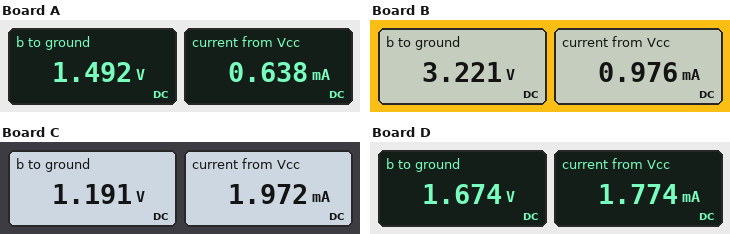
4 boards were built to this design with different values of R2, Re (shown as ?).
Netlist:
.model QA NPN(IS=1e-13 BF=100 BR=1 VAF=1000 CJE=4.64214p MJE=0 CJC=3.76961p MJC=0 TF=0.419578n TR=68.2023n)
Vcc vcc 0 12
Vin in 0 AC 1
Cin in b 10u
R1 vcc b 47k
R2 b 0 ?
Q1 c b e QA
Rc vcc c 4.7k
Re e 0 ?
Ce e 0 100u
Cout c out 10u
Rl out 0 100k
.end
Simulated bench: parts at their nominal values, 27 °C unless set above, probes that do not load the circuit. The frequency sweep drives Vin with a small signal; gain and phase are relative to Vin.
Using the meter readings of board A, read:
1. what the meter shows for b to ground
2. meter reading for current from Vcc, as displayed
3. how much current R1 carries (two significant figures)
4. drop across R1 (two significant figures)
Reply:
1.492 V
0.638 mA
220 µA
11 V
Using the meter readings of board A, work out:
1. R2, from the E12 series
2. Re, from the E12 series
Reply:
6.8 kΩ
2.2 kΩ
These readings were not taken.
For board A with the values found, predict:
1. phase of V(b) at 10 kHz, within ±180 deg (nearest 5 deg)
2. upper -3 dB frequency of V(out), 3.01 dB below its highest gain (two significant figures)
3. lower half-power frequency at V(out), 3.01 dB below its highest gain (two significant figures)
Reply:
0 deg
9.4 MHz
29 Hz
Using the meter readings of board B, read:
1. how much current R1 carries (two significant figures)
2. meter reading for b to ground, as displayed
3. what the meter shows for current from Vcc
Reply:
190 µA
3.221 V
0.976 mA
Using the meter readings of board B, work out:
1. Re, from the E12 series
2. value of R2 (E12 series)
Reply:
3.3 kΩ
18 kΩ
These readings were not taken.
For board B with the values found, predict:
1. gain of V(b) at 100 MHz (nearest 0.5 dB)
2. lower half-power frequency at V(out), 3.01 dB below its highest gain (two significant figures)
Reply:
0 dB
54 Hz
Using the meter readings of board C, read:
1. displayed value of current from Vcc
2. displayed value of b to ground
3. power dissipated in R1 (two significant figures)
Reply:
1.972 mA
1.191 V
2.5 mW
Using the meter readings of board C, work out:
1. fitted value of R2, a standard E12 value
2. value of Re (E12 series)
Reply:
5.6 kΩ
330 Ω
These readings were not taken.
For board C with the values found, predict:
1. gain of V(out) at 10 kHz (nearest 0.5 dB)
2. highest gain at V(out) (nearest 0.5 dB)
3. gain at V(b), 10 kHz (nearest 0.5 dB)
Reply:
49.5 dB
49.5 dB
0 dB
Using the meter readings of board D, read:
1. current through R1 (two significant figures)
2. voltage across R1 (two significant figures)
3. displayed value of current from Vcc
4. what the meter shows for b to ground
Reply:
220 µA
10 V
1.774 mA
1.674 V
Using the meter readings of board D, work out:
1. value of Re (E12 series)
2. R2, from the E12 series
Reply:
680 Ω
8.2 kΩ
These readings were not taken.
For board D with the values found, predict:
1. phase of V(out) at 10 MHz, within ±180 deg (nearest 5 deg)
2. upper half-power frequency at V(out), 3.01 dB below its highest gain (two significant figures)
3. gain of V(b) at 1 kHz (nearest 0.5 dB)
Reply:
135 deg
9.5 MHz
0 dB
